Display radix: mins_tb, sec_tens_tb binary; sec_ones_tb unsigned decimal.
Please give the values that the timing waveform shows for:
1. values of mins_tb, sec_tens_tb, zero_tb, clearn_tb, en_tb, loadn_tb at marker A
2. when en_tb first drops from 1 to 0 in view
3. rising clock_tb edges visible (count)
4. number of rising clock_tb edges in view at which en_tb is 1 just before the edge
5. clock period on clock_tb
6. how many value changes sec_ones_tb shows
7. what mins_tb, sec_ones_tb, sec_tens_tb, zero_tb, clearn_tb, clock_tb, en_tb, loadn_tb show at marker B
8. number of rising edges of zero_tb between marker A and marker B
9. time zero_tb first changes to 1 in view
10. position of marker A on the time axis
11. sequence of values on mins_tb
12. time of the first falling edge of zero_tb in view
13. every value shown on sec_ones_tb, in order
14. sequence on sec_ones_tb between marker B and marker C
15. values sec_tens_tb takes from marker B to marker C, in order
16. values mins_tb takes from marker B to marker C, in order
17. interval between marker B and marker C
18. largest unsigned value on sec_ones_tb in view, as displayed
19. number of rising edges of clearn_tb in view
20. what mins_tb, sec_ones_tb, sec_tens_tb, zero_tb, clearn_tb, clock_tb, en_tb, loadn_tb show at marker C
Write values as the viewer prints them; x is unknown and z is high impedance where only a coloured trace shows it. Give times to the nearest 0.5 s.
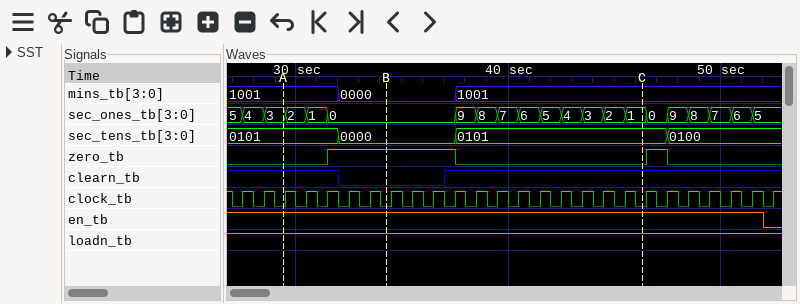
mins_tb=1001, sec_tens_tb=0101, zero_tb=0, clearn_tb=1, en_tb=1, loadn_tb=1
52 s
26
25
1 s
20
mins_tb=0000, sec_ones_tb=0, sec_tens_tb=0000, zero_tb=1, clearn_tb=0, clock_tb=0, en_tb=1, loadn_tb=1
1
31.5 s
29.5 s
1001, 0000, 1001
37.5 s
5, 4, 3, 2, 1, 0, 9, 8, 7, 6, 5, 4, 3, 2, 1, 0, 9, 8, 7, 6, 5
0, 9, 8, 7, 6, 5, 4, 3, 2, 1
0000, 0101
0000, 1001
12 s
9
1
mins_tb=1001, sec_ones_tb=1, sec_tens_tb=0101, zero_tb=0, clearn_tb=1, clock_tb=0, en_tb=1, loadn_tb=1
